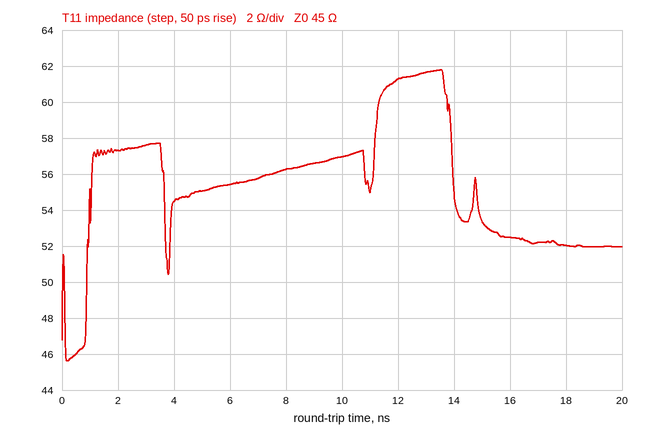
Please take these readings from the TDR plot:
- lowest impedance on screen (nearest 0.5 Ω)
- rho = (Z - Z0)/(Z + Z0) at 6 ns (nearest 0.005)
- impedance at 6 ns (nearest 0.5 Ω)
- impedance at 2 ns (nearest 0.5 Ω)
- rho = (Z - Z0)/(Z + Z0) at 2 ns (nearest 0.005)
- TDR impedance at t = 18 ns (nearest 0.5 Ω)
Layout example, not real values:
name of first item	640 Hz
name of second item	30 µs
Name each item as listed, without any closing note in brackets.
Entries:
lowest impedance on screen	45.5 Ω
rho = (Z - Z0)/(Z + Z0) at 6 ns	+0.105
impedance at 6 ns	55.5 Ω
impedance at 2 ns	57.5 Ω
rho = (Z - Z0)/(Z + Z0) at 2 ns	+0.120
TDR impedance at t = 18 ns	52.0 Ω
